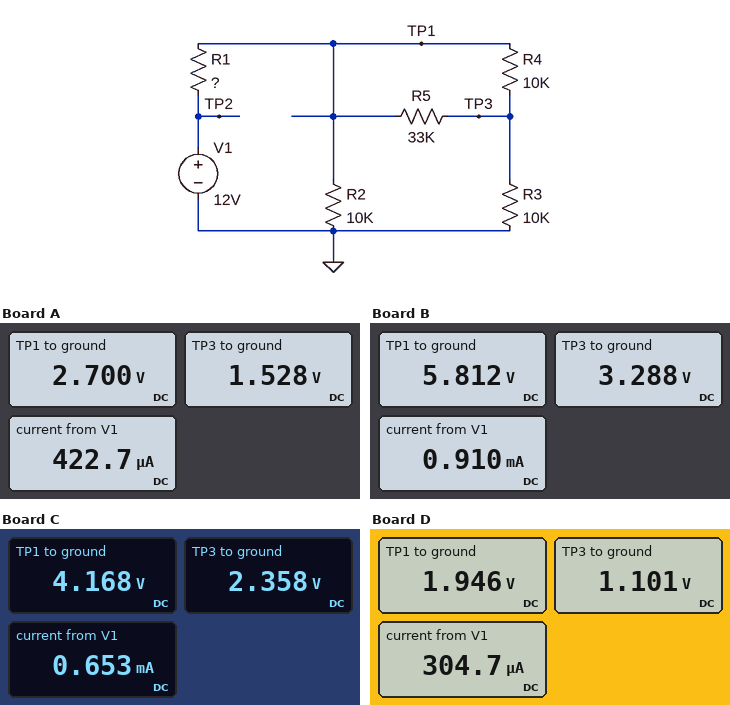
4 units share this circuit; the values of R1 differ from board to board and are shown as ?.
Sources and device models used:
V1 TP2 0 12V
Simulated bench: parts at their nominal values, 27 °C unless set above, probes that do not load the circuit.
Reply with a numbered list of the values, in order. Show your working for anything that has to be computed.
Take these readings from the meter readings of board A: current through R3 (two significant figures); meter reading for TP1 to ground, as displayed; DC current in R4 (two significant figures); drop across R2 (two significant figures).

1. (1.528 V) / 10 kΩ = 150 µA
2. 2.700 V
3. (2.7 V - 1.528 V) / 10 kΩ = 120 µA
4. 2.7 V = 2.7 V
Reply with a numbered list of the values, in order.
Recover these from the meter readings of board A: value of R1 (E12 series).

1. 22 kΩ
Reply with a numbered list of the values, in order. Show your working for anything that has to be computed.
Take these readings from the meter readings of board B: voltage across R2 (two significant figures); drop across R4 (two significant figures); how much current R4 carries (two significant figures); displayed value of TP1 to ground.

1. 5.812 V = 5.8 V
2. 5.812 V - 3.288 V = 2.5 V
3. (5.812 V - 3.288 V) / 10 kΩ = 250 µA
4. 5.812 V
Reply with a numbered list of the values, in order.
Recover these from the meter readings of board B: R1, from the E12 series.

1. 6.8 kΩ
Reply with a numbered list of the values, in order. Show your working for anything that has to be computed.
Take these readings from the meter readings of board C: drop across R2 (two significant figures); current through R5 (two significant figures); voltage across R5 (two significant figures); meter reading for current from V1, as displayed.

1. 4.168 V = 4.2 V
2. (4.168 V - 2.358 V) / 33 kΩ = 55 µA
3. 4.168 V - 2.358 V = 1.8 V
4. 0.653 mA
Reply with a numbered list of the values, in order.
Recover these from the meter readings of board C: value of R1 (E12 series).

1. 12 kΩ
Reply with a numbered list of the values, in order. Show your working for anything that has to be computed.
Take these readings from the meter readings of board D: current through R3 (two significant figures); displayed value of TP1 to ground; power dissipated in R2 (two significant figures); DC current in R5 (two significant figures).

1. (1.101 V) / 10 kΩ = 110 µA
2. 1.946 V
3. (1.946 V)^2 / 10 kΩ = 380 µW
4. (1.946 V - 1.101 V) / 33 kΩ = 26 µA
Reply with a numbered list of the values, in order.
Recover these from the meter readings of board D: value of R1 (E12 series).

1. 33 kΩ
